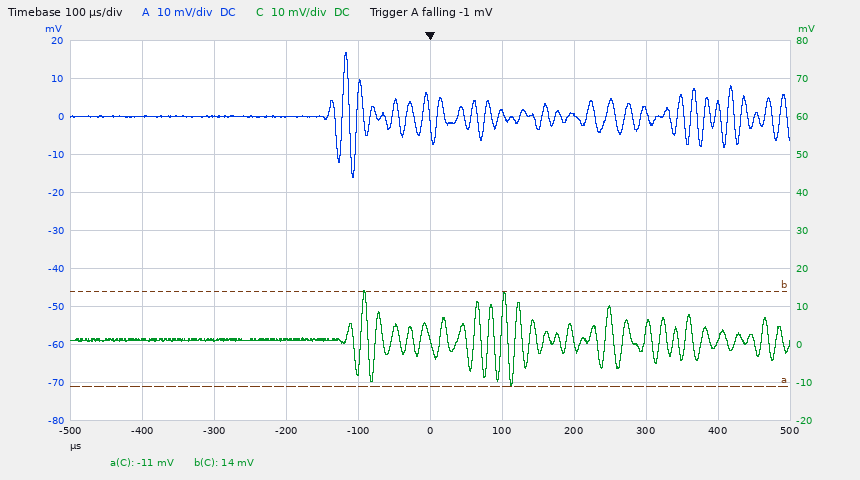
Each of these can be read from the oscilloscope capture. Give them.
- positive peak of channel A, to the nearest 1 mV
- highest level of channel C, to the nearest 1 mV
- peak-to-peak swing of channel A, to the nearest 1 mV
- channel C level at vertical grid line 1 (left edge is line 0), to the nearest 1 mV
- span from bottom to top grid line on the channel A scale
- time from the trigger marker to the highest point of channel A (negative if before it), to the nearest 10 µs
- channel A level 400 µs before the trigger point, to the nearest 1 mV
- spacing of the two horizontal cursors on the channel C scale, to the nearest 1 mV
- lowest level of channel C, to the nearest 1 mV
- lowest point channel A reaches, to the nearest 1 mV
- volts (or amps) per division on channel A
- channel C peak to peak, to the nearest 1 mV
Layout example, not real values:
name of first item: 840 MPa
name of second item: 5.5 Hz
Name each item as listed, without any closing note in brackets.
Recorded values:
positive peak of channel A, to the nearest 1 mV: 17 mV
highest level of channel C, to the nearest 1 mV: 14 mV
peak-to-peak swing of channel A, to the nearest 1 mV: 33 mV
channel C level at vertical grid line 1 (left edge is line 0), to the nearest 1 mV: 1 mV
span from bottom to top grid line on the channel A scale: 100 mV
time from the trigger marker to the highest point of channel A (negative if before it), to the nearest 10 µs: -120 µs
channel A level 400 µs before the trigger point, to the nearest 1 mV: 0 mV
spacing of the two horizontal cursors on the channel C scale, to the nearest 1 mV: 25 mV
lowest level of channel C, to the nearest 1 mV: -11 mV
lowest point channel A reaches, to the nearest 1 mV: -16 mV
volts (or amps) per division on channel A: 10 mV
channel C peak to peak, to the nearest 1 mV: 25 mV
